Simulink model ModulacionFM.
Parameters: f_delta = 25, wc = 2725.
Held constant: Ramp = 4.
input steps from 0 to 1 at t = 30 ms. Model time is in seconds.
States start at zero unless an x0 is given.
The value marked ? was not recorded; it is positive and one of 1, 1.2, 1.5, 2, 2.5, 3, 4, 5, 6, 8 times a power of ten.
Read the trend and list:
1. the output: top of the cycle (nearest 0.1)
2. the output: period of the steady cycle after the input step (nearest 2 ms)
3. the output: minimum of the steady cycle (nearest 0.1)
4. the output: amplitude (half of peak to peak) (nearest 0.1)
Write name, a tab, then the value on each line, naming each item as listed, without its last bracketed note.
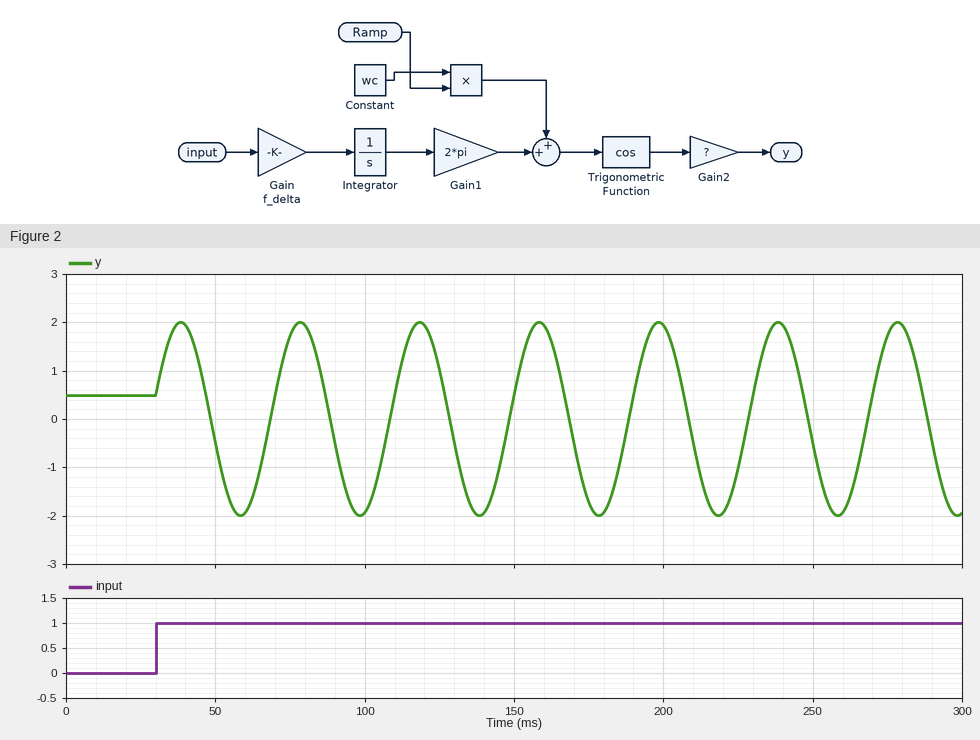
the output: top of the cycle	2.0
the output: period of the steady cycle after the input step	40 ms
the output: minimum of the steady cycle	-2.0
the output: amplitude (half of peak to peak)	2.0
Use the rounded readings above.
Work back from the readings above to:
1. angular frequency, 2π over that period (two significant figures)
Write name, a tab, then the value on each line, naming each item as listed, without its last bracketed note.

angular frequency, 2π over that period	0.16 rad/ms
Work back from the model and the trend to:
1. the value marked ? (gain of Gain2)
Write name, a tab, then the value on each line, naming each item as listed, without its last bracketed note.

the value marked ?	2
